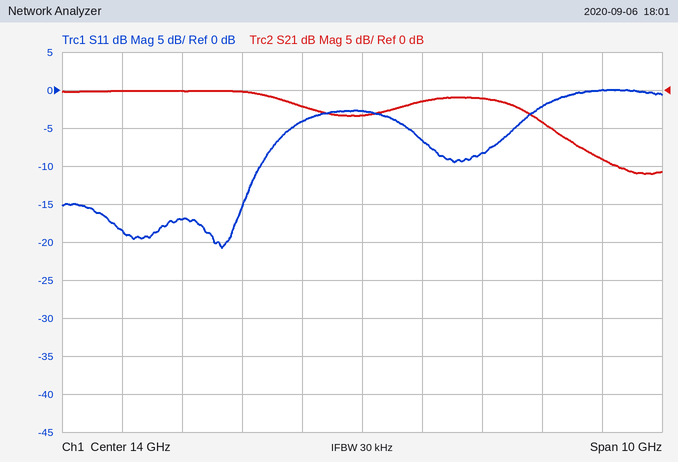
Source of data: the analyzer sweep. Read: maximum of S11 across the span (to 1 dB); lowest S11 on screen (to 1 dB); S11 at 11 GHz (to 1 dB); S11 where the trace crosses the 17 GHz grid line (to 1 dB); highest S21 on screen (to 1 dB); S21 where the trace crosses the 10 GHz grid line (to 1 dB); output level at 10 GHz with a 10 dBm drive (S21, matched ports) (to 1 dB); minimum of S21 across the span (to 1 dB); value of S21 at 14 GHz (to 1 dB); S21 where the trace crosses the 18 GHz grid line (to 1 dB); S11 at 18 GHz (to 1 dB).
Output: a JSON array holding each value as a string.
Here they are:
["0 dB", "-21 dB", "-17 dB", "-2 dB", "0 dB", "0 dB", "10 dBm", "-11 dB", "-3 dB", "-9 dB", "0 dB"]
